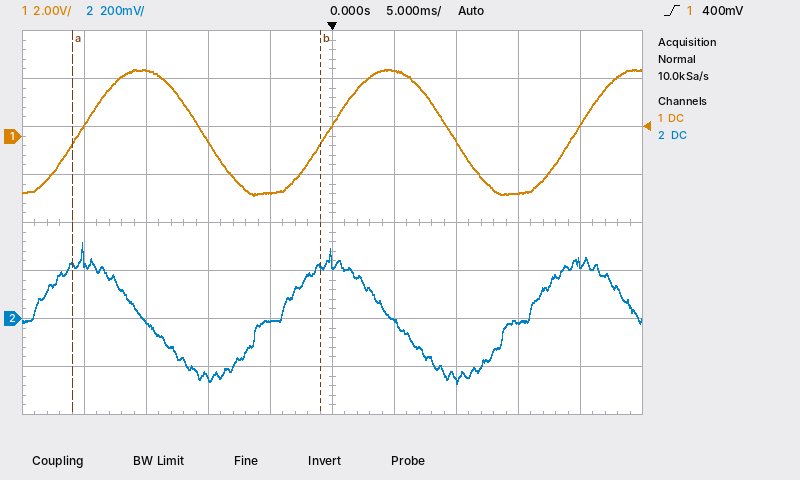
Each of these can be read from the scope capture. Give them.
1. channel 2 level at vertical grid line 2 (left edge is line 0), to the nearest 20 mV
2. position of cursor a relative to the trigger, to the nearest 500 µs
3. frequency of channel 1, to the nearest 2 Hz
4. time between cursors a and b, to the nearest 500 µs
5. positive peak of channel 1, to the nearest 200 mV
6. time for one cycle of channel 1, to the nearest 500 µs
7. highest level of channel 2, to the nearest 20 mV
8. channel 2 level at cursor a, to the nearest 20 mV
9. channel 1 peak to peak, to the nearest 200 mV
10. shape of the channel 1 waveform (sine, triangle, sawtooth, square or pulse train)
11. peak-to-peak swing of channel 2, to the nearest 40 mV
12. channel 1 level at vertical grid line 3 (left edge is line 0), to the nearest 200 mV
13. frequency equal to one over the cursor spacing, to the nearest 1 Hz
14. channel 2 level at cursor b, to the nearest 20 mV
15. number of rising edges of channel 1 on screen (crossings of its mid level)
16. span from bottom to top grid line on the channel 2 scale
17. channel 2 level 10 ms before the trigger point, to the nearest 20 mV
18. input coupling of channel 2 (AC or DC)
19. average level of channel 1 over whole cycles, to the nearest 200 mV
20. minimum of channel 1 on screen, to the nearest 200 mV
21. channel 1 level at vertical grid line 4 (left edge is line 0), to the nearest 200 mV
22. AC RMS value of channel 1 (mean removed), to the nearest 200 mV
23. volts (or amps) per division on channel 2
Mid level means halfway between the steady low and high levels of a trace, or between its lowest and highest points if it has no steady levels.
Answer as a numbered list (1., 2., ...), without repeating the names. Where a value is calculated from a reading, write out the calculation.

1. -20 mV
2. -21.0 ms
3. 1 / 20.0 ms ≈ 50 Hz
4. 20.0 ms
5. 2.8 V
6. 20.0 ms
7. 320 mV
8. 220 mV
9. 2.8 V − (-2.4 V) = 5.2 V
10. sine
11. 600 mV
12. -200 mV
13. 1 / 20.0 ms ≈ 50 Hz
14. 220 mV
15. 3
16. 1.6 V
17. -240 mV
18. DC
19. (2.8 V + (-2.4 V)) / 2 ≈ 200 mV
20. -2.4 V
21. -2.4 V
22. 5.2 V / (2√2) ≈ 1.8 V
23. 200 mV
